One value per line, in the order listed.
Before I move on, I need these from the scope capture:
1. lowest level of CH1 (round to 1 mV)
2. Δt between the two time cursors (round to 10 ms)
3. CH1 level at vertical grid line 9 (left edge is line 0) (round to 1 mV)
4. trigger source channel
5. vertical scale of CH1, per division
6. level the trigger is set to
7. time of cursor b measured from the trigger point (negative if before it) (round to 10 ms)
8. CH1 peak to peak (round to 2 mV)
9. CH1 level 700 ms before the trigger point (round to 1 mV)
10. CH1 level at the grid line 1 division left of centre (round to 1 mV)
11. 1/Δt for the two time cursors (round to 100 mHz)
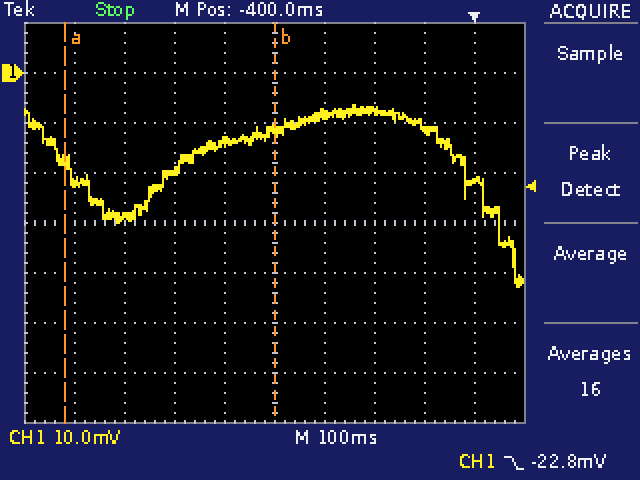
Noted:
-43 mV
420 ms
-22 mV
CH1
10 mV
-22.8 mV
-400 ms
36 mV
-29 mV
-14 mV
2.4 Hz
